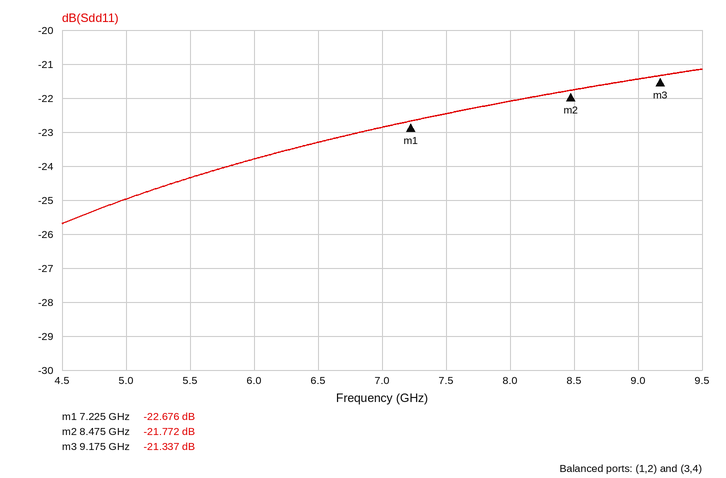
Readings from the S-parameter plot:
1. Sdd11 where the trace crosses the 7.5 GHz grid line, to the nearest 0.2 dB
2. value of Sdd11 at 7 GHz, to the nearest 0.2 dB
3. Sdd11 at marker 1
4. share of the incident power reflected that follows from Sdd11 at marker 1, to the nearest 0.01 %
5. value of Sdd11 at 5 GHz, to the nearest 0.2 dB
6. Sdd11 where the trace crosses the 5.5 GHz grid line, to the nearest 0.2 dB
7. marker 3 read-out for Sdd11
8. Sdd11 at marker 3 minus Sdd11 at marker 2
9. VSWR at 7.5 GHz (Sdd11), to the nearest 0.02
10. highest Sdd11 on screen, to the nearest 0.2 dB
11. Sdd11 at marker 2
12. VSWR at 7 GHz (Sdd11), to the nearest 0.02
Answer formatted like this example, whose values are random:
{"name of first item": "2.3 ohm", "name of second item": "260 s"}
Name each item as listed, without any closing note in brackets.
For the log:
{"Sdd11 where the trace crosses the 7.5 GHz grid line, to the nearest 0.2 dB": "-22.4 dB", "value of Sdd11 at 7 GHz, to the nearest 0.2 dB": "-22.8 dB", "Sdd11 at marker 1": "-22.676 dB", "share of the incident power reflected that follows from Sdd11 at marker 1, to the nearest 0.01 %": "0.54 %", "value of Sdd11 at 5 GHz, to the nearest 0.2 dB": "-25.0 dB", "Sdd11 where the trace crosses the 5.5 GHz grid line, to the nearest 0.2 dB": "-24.4 dB", "marker 3 read-out for Sdd11": "-21.337 dB", "Sdd11 at marker 3 minus Sdd11 at marker 2": "0.435 dB", "VSWR at 7.5 GHz (Sdd11), to the nearest 0.02": "1.16", "highest Sdd11 on screen, to the nearest 0.2 dB": "-21.2 dB", "Sdd11 at marker 2": "-21.772 dB", "VSWR at 7 GHz (Sdd11), to the nearest 0.02": "1.16"}
